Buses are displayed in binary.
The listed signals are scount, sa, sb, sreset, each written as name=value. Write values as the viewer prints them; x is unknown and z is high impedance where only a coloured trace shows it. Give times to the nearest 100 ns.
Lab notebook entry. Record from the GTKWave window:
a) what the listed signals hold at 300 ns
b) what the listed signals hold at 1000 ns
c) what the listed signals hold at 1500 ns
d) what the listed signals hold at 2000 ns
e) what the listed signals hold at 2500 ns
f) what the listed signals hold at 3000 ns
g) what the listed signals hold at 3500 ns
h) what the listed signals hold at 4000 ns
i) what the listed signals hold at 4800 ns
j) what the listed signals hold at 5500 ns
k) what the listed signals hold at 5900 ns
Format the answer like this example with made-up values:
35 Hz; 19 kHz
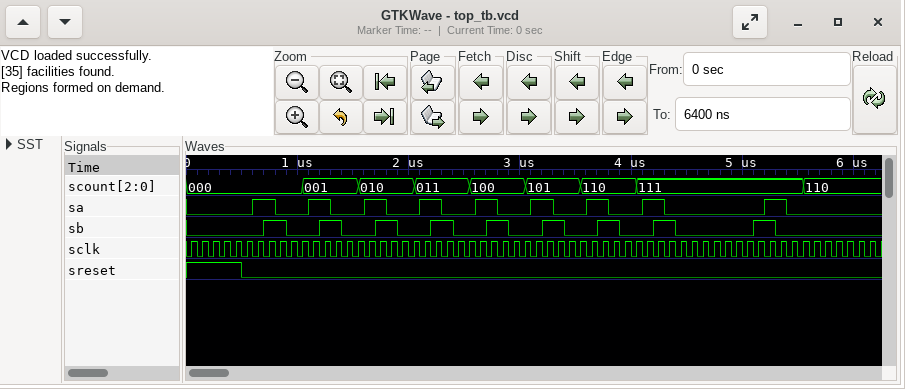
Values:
scount=000, sa=0, sb=0, sreset=1; scount=000, sa=0, sb=0, sreset=0; scount=001, sa=0, sb=0, sreset=0; scount=010, sa=0, sb=0, sreset=0; scount=011, sa=0, sb=0, sreset=0; scount=100, sa=0, sb=0, sreset=0; scount=101, sa=0, sb=0, sreset=0; scount=110, sa=0, sb=0, sreset=0; scount=111, sa=0, sb=0, sreset=0; scount=111, sa=0, sb=0, sreset=0; scount=110, sa=0, sb=0, sreset=0
